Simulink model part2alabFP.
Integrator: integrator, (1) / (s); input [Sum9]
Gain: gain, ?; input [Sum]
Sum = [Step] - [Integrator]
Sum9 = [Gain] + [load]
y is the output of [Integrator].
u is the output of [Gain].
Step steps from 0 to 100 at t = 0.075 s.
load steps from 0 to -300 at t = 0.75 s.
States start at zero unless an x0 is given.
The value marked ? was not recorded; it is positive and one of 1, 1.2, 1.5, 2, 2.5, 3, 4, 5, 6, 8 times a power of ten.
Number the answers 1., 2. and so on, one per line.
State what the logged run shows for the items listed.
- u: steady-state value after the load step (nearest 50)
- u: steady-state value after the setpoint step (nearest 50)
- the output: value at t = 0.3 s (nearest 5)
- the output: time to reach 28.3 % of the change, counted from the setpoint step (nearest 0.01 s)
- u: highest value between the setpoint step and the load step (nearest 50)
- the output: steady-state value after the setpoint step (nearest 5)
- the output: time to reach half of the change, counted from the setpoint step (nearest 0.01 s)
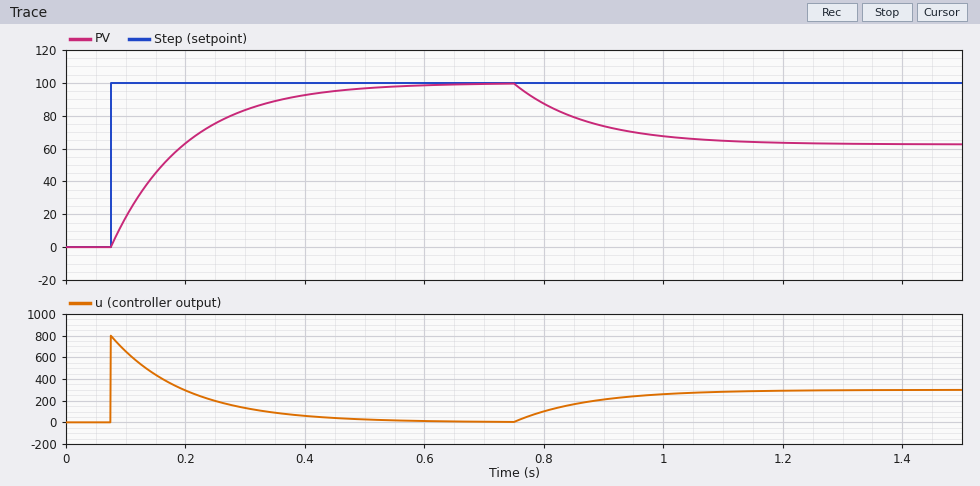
1. 300
2. 0
3. 85
4. 0.04 s
5. 800
6. 100
7. 0.09 s
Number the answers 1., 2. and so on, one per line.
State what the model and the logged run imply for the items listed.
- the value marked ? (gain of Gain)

1. 8
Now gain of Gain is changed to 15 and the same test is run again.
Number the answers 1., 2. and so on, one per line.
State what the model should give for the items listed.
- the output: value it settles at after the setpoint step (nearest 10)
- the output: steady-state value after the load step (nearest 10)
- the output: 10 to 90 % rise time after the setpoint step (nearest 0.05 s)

1. 100
2. 80
3. 0.15 s
